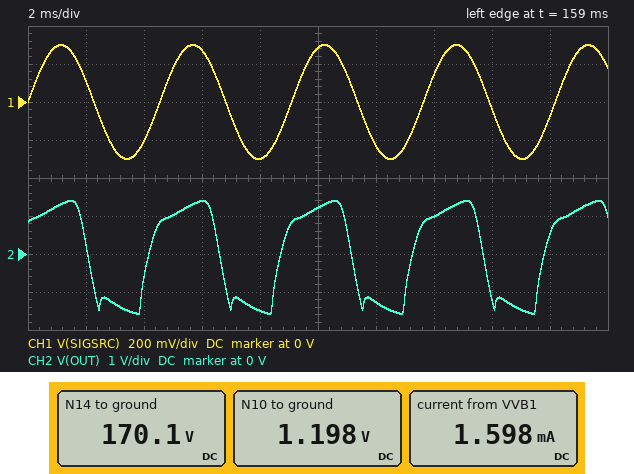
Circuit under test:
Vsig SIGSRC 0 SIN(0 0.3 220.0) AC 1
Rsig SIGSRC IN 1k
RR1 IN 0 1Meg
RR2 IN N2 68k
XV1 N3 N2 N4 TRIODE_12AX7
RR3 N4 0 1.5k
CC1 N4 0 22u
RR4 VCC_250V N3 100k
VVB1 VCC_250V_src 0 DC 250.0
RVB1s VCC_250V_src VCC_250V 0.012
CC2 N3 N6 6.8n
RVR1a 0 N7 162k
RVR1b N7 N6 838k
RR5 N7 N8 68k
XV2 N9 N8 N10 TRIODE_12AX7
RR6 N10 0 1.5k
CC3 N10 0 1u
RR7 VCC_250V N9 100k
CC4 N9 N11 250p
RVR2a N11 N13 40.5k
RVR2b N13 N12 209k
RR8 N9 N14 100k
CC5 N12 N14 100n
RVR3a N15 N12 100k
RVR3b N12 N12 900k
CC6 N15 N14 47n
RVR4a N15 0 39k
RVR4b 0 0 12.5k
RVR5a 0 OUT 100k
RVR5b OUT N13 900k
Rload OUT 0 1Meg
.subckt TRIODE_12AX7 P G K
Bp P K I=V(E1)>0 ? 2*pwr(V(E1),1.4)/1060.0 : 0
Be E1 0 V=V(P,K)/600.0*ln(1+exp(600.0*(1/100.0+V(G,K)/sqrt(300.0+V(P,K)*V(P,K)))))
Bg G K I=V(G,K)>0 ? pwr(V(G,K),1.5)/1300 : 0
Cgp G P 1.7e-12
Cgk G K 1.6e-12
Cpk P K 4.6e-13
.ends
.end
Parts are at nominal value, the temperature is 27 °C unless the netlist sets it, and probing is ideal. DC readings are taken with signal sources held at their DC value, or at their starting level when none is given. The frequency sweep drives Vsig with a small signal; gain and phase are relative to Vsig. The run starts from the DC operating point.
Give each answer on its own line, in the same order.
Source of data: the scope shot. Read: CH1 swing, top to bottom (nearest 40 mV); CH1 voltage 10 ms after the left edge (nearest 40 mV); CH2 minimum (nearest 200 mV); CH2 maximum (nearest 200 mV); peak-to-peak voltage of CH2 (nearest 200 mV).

600 mV
280 mV
-1.6 V
1.4 V
3.0 V
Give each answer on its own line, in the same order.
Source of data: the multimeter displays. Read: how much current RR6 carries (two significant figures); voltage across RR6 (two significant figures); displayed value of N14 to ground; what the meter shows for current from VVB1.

800 µA
1.2 V
170.1 V
1.598 mA
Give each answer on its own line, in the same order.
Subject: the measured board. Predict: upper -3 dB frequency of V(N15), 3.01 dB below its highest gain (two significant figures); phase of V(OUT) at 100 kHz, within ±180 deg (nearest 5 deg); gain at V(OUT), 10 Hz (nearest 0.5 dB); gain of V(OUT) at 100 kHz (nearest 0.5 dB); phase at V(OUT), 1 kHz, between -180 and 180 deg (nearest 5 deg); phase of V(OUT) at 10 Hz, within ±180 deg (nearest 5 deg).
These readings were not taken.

10 kHz
-160 deg
8.5 dB
-3.0 dB
30 deg
105 deg
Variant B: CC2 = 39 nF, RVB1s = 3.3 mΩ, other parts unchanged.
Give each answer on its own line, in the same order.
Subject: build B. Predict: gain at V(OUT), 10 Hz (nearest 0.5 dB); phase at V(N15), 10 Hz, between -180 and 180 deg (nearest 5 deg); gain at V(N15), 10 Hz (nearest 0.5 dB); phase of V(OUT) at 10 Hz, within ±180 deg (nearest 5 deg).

15.5 dB
70 deg
29.5 dB
60 deg
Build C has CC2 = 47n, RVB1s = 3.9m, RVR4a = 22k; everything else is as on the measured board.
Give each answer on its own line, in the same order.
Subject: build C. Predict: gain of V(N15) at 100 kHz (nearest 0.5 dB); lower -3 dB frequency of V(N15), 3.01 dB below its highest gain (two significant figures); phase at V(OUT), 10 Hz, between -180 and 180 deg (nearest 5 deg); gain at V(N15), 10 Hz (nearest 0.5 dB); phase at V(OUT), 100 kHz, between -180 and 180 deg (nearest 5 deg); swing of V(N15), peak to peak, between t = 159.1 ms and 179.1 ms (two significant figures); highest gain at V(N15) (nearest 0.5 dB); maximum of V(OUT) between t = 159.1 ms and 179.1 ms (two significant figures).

6.5 dB
240 Hz
60 deg
25.5 dB
-160 deg
20 V
38.5 dB
1.1 V
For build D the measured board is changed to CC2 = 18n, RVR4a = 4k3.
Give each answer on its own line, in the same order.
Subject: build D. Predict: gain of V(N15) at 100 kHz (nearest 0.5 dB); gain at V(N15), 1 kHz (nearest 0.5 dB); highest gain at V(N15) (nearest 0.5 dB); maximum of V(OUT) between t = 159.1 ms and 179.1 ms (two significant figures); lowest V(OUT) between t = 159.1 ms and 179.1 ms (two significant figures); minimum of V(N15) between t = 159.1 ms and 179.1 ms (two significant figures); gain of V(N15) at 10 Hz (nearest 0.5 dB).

-6.0 dB
25.0 dB
25.5 dB
680 mV
-760 mV
-2.5 V
10.0 dB
